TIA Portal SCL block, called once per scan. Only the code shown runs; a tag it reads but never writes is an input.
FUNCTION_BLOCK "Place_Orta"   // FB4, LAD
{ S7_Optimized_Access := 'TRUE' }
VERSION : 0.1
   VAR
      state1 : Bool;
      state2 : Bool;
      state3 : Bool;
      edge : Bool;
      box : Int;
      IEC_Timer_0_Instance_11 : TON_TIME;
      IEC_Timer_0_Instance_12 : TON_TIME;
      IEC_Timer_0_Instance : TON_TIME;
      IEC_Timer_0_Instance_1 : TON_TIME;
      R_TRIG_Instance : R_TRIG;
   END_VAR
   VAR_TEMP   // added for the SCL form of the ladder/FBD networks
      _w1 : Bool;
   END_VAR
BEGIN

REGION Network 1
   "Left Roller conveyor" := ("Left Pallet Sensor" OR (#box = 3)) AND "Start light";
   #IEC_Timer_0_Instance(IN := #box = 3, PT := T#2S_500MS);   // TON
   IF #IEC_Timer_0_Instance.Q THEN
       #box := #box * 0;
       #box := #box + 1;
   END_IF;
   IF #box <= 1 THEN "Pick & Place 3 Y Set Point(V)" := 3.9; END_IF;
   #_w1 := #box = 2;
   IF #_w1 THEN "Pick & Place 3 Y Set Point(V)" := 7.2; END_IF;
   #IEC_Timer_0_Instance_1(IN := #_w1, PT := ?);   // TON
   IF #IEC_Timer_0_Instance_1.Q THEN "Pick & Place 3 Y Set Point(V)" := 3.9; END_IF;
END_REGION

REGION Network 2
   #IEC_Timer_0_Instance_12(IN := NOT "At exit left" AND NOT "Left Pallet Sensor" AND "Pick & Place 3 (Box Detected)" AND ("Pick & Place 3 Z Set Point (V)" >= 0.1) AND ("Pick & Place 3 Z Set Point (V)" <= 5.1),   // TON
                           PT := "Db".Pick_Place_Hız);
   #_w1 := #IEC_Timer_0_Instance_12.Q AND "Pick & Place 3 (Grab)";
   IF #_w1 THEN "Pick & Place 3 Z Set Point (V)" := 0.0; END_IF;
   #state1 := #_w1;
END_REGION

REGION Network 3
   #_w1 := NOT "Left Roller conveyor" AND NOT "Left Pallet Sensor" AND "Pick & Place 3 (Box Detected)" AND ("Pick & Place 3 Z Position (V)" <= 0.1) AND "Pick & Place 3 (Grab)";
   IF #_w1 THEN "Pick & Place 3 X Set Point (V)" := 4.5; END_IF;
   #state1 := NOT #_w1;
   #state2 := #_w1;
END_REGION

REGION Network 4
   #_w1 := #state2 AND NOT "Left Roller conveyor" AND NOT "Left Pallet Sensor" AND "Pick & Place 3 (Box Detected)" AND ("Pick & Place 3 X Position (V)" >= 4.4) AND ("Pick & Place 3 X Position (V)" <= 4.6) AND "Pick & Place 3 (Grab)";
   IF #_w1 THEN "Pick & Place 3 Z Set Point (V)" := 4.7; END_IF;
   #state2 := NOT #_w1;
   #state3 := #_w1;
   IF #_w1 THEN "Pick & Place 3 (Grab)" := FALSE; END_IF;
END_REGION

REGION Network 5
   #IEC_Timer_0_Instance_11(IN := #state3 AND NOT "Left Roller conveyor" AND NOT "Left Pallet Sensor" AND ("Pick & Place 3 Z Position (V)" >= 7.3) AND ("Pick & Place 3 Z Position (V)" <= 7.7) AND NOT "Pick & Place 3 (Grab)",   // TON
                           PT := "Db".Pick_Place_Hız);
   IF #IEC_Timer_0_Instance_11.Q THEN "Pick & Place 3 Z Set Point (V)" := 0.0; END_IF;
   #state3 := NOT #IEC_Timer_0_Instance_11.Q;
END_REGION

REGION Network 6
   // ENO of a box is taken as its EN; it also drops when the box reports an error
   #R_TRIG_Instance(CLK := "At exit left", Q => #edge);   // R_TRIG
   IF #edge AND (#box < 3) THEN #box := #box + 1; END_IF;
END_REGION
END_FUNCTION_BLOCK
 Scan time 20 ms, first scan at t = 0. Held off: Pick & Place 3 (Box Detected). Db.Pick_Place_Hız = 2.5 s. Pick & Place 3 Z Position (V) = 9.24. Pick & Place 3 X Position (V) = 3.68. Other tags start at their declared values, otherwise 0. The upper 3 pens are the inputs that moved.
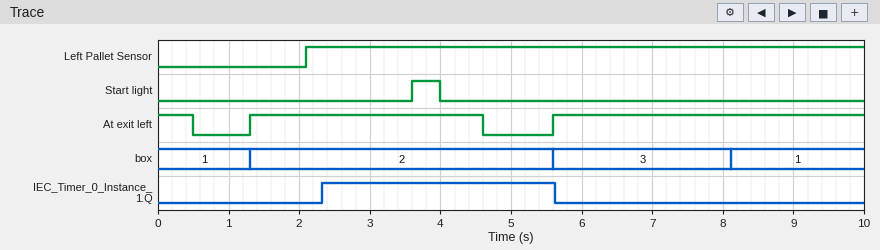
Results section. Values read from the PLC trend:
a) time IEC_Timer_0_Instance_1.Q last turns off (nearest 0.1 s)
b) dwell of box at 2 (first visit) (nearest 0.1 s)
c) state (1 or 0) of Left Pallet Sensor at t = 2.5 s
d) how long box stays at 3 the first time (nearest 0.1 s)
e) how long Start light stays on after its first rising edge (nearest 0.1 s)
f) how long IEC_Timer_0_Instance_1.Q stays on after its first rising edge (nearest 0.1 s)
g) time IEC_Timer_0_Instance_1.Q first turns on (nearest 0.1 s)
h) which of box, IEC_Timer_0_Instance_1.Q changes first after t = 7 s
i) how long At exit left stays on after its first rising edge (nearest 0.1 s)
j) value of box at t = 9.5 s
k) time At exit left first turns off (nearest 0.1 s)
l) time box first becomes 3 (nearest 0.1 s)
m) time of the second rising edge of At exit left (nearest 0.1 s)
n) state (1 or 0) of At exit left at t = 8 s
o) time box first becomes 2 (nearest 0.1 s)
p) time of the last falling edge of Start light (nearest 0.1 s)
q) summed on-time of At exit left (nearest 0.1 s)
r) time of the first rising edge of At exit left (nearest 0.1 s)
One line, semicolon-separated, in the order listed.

5.6 s; 4.3 s; 1; 2.5 s; 0.4 s; 3.3 s; 2.3 s; box; 3.3 s; 1; 0.5 s; 5.6 s; 5.6 s; 1; 1.3 s; 4.0 s; 8.2 s; 1.3 s
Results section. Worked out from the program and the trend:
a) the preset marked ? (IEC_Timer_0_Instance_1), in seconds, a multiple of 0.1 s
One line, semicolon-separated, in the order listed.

1.0 s
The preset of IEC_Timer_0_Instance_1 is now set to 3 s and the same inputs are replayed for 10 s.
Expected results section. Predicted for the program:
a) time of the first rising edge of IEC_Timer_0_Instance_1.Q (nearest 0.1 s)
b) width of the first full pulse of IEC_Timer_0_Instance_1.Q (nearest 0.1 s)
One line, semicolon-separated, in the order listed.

4.3 s; 1.3 s
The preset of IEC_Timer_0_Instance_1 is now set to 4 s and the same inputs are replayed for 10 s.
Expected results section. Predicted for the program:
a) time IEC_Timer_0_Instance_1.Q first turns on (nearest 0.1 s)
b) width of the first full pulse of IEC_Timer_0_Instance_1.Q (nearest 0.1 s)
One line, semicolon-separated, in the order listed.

5.3 s; 0.3 s
